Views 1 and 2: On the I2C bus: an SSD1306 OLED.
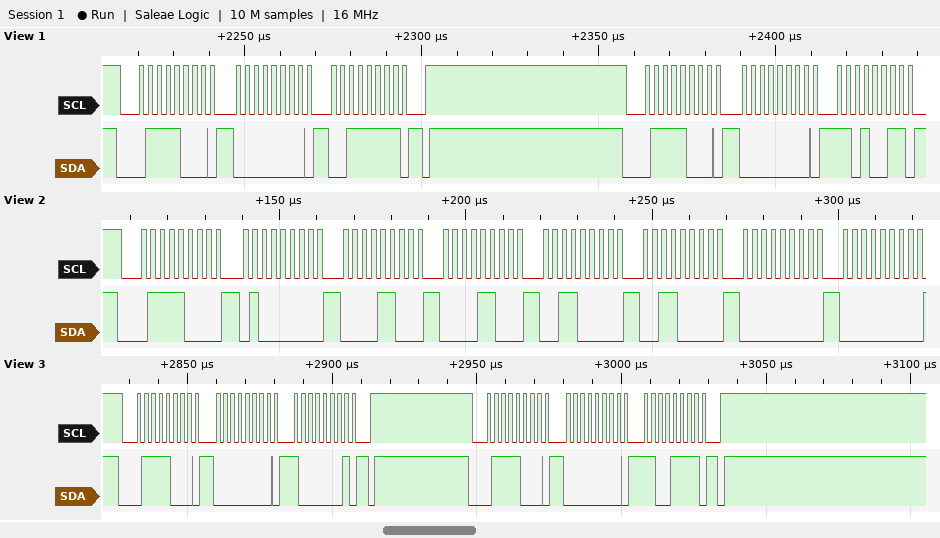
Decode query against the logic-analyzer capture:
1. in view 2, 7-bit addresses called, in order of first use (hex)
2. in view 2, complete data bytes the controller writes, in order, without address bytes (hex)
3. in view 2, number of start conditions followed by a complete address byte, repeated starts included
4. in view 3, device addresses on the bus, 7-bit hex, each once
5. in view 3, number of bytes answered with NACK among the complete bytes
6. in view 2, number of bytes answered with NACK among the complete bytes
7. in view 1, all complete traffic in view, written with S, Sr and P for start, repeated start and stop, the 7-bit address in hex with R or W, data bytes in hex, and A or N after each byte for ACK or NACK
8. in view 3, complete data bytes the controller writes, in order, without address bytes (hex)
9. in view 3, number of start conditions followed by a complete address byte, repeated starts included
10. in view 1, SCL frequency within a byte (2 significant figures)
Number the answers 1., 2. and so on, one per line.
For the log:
1. 0x3C
2. 40 0C 0C 30 30 00 00
3. 1
4. 0x3C
5. 0
6. 0
7. S 3CW A 00 A 3F A P S 3CW A 00 A D3 A
8. 00 81 00 CF
9. 2
10. 400 kHz
